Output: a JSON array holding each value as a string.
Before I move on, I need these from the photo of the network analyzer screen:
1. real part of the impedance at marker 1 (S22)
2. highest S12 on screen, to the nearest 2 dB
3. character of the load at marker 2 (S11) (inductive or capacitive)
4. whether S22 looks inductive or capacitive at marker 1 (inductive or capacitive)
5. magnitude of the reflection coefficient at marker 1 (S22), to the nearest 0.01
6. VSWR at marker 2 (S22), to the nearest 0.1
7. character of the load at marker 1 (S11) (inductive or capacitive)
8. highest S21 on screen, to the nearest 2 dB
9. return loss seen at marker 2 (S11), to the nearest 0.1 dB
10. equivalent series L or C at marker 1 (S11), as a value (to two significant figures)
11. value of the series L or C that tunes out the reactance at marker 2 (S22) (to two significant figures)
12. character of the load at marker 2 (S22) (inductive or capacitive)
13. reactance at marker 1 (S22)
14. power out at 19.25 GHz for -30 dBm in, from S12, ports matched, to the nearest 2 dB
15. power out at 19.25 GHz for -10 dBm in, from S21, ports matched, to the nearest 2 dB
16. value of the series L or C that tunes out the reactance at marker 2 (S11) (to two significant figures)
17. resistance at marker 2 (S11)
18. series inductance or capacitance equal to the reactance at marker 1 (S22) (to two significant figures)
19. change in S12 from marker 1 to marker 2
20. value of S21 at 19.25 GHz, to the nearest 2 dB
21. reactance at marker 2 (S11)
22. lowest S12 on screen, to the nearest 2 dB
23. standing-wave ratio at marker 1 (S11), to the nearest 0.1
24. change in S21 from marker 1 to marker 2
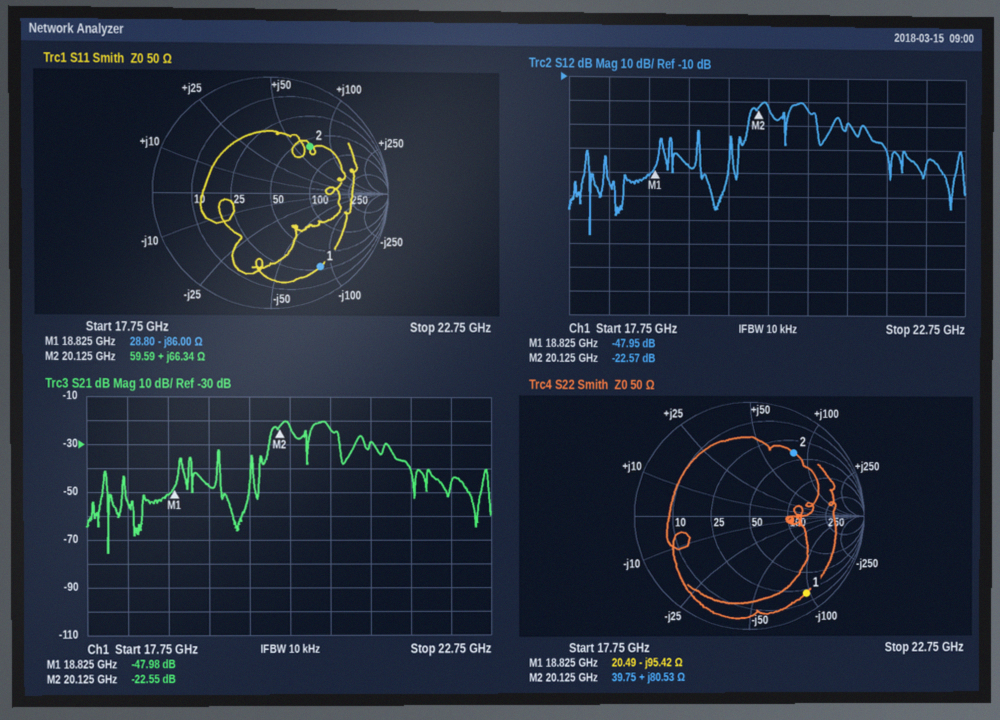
["20.49 Ω", "-20 dB", "inductive", "capacitive", "0.84", "5.1", "capacitive", "-20 dB", "5.6 dB", "98 fF", "98 fF", "inductive", "-95.42 Ω", "-78 dBm", "-58 dBm", "120 fF", "59.59 Ω", "89 fF", "25.38 dB", "-48 dB", "+66.34 Ω", "-76 dB", "7.3", "25.43 dB"]
